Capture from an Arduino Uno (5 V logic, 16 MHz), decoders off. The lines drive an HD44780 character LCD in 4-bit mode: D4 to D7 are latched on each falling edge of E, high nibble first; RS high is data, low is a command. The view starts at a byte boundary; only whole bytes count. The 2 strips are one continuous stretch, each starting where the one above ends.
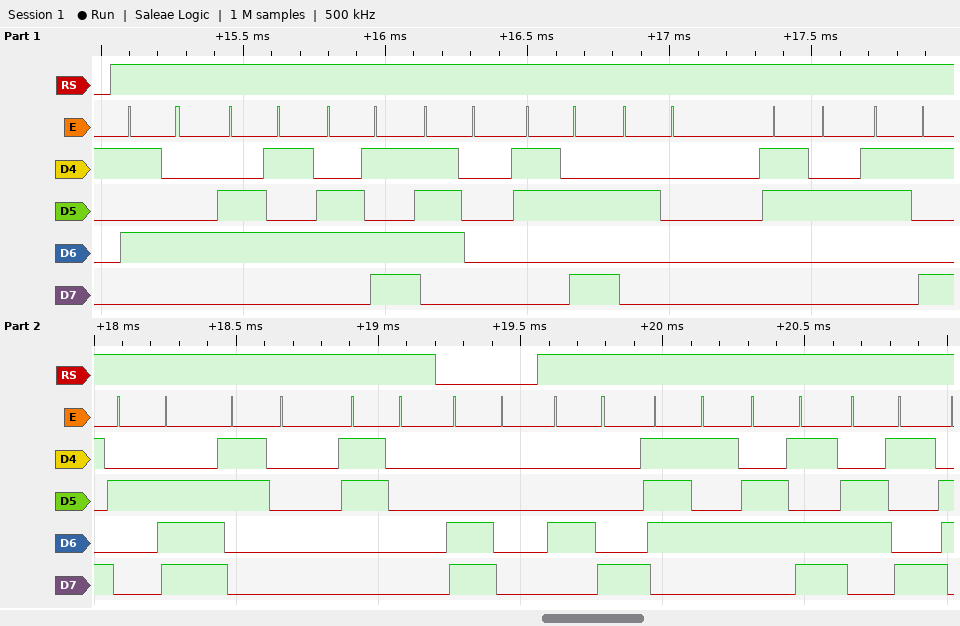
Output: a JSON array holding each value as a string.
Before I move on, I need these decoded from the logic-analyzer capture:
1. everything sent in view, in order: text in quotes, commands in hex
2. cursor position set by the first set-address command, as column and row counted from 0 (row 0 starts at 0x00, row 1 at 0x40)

["\"Temp: 29.00\" 0xC0 \"Humi\"", "column 0, row 1"]
